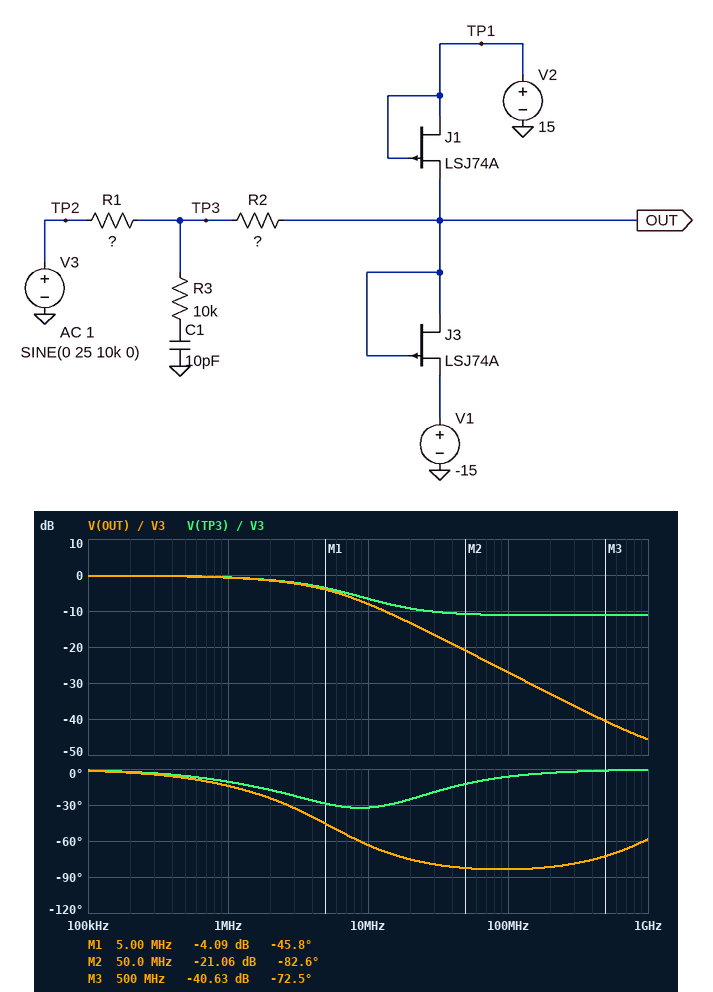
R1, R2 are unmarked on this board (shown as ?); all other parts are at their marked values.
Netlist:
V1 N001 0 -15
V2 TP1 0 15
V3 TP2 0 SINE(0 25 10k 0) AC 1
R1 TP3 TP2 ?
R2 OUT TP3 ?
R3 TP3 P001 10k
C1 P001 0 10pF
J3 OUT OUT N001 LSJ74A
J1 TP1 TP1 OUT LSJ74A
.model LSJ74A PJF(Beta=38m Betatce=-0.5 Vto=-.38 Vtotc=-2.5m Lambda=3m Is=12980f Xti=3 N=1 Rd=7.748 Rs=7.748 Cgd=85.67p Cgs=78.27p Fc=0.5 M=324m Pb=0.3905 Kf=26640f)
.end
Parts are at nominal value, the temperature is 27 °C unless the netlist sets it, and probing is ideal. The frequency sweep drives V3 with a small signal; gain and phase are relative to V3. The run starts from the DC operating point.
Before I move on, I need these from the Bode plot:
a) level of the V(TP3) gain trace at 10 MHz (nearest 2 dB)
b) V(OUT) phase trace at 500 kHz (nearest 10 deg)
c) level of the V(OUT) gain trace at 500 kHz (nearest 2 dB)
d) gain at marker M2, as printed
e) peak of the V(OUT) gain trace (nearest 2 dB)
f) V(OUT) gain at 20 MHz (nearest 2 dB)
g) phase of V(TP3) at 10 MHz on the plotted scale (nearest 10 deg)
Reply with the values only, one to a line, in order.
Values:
-6 dB
-10 deg
0 dB
-21.06 dB
0 dB
-14 dB
-30 deg
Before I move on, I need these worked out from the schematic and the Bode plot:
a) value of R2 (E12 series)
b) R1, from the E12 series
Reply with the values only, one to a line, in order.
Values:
390 Ω
1 kΩ
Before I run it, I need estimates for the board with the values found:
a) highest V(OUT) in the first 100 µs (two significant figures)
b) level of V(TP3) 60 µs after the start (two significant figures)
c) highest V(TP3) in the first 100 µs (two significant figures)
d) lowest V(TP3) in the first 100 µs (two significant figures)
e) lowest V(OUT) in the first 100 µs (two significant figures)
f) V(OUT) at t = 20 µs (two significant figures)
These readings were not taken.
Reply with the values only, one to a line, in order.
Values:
15 V
-14 V
18 V
-18 V
-15 V
15 V
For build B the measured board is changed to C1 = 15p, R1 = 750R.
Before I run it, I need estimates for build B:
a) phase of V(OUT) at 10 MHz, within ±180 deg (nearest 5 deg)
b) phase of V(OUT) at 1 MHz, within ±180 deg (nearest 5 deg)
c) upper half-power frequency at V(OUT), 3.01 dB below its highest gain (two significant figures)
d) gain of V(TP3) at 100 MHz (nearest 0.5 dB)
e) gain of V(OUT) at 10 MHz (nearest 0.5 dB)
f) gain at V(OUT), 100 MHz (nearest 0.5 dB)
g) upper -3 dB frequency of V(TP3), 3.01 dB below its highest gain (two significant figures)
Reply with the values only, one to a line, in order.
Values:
-60 deg
-10 deg
5.1 MHz
-9.5 dB
-6.5 dB
-25.5 dB
5.8 MHz
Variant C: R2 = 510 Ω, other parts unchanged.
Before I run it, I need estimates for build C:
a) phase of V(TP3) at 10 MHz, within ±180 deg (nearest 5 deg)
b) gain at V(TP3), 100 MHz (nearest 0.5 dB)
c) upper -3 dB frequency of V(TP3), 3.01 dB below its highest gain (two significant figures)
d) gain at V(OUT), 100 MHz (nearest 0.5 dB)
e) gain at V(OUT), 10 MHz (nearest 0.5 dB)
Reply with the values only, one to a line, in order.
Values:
-25 deg
-9.5 dB
4.2 MHz
-28.0 dB
-8.5 dB
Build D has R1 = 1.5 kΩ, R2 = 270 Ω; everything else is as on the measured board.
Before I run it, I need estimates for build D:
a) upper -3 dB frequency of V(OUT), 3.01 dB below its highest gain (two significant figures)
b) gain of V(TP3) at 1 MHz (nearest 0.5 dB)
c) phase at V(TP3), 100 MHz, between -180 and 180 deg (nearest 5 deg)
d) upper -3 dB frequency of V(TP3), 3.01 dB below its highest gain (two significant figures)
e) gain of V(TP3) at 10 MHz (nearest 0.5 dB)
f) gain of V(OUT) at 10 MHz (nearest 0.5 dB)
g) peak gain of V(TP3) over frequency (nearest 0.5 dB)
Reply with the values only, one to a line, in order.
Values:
3.0 MHz
-1.0 dB
-10 deg
3.1 MHz
-9.0 dB
-10.0 dB
-0.5 dB
